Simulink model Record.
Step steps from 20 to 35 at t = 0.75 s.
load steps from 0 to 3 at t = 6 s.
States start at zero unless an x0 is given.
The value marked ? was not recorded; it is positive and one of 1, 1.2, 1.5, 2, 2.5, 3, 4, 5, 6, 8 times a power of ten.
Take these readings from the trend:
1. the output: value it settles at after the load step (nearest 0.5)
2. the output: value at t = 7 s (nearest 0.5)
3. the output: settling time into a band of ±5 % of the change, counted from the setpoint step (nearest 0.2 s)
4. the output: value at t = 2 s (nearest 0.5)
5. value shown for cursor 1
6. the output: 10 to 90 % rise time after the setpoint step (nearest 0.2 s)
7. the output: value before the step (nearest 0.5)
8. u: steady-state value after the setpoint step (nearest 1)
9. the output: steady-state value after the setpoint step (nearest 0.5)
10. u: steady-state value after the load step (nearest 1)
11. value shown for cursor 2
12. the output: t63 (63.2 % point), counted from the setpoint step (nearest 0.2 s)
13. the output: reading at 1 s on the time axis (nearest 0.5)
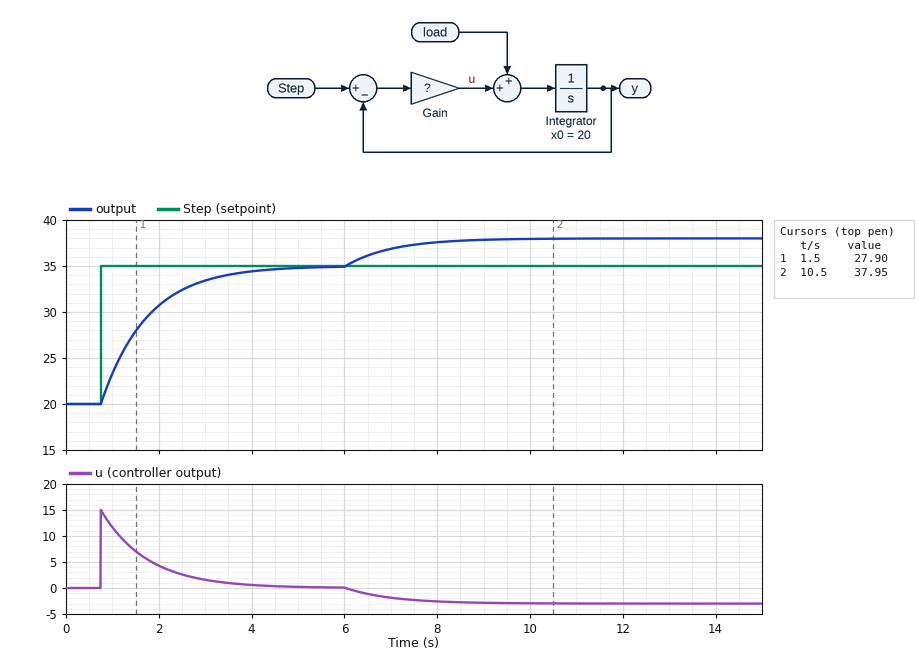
38.0
37.0
3.0 s
30.5
27.90
2.2 s
20.0
0
35.0
-3
37.95
1.0 s
23.5
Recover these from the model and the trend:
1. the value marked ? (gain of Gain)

1
